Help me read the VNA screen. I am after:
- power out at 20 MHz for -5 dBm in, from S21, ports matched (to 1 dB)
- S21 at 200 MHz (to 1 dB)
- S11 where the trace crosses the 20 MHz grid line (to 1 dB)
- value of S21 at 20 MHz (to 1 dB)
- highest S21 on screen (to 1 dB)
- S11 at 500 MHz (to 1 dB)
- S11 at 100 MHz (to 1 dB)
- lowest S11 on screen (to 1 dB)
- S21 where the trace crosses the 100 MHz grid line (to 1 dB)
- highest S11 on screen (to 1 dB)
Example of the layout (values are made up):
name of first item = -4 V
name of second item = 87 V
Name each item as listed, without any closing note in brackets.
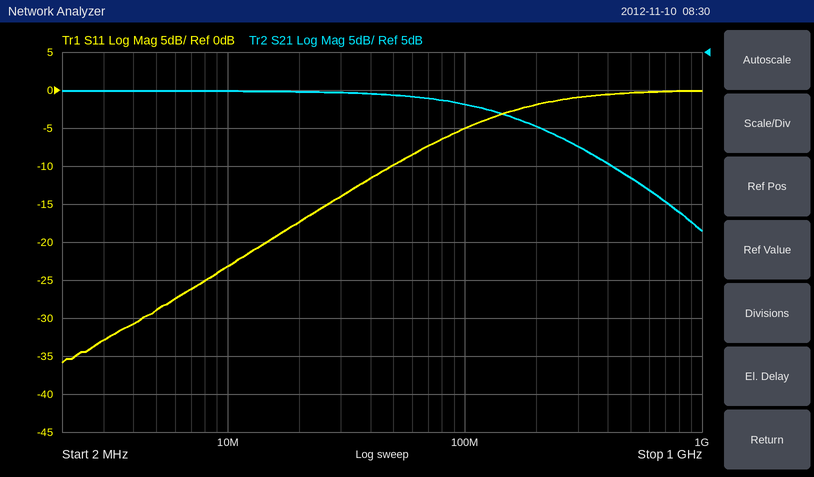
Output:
power out at 20 MHz for -5 dBm in, from S21, ports matched = -5 dBm
S21 at 200 MHz = -5 dB
S11 where the trace crosses the 20 MHz grid line = -17 dB
value of S21 at 20 MHz = 0 dB
highest S21 on screen = 0 dB
S11 at 500 MHz = 0 dB
S11 at 100 MHz = -5 dB
lowest S11 on screen = -36 dB
S21 where the trace crosses the 100 MHz grid line = -2 dB
highest S11 on screen = 0 dB
